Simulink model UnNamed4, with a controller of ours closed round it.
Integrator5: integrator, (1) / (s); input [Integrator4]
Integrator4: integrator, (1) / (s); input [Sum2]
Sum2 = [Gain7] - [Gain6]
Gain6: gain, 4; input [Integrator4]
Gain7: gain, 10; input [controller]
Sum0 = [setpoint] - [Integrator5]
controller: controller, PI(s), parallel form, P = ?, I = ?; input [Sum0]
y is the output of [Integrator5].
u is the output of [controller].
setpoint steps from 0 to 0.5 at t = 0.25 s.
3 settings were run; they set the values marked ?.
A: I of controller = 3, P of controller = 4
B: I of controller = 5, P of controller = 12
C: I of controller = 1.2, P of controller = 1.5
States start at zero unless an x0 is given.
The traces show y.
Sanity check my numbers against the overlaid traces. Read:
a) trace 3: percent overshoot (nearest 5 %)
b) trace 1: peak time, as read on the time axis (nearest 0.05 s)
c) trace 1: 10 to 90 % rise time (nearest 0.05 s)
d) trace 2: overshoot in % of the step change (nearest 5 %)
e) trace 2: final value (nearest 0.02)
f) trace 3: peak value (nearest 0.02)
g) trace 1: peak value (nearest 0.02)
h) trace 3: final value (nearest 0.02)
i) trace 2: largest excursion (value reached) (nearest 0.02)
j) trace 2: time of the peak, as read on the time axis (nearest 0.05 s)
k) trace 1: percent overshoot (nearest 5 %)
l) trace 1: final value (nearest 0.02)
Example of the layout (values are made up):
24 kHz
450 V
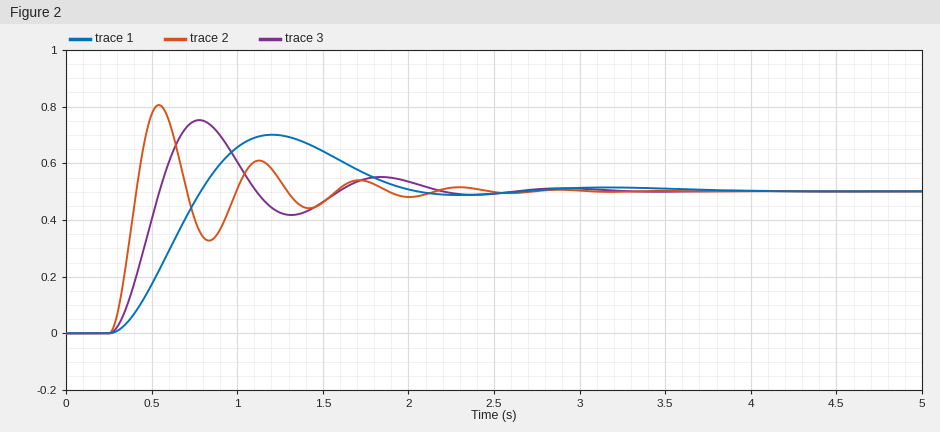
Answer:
50 %
1.20 s
0.35 s
60 %
0.50
0.76
0.70
0.50
0.80
0.55 s
40 %
0.50
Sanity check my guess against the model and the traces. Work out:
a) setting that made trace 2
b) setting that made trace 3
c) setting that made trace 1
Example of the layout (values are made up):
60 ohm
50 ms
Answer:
B
A
C
